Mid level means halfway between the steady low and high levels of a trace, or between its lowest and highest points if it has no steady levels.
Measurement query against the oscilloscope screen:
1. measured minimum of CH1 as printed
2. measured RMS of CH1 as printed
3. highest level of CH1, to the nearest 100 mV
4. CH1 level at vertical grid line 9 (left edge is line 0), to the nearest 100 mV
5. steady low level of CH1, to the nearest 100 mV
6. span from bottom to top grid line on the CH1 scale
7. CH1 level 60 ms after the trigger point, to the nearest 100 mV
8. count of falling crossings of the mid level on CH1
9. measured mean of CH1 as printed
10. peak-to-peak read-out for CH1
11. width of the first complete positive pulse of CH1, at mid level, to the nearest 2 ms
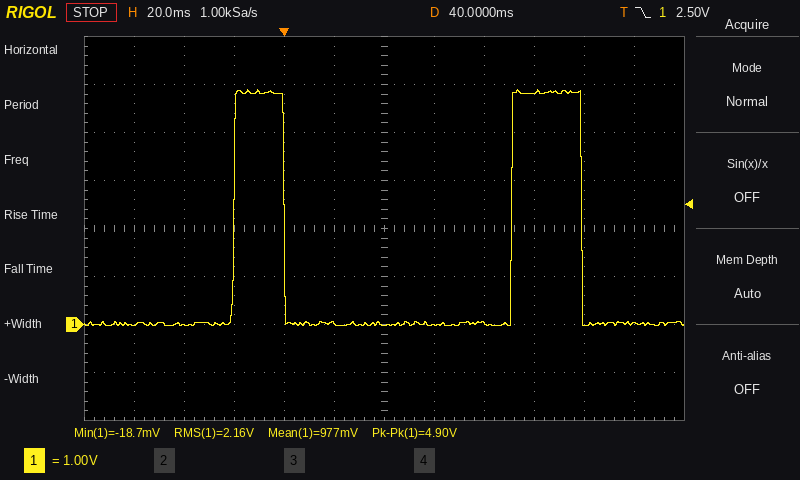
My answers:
-18.7 mV
2.16 V
4.9 V
4.8 V
0.0 V
8 V
0.0 V
2
977 mV
4.90 V
20 ms
